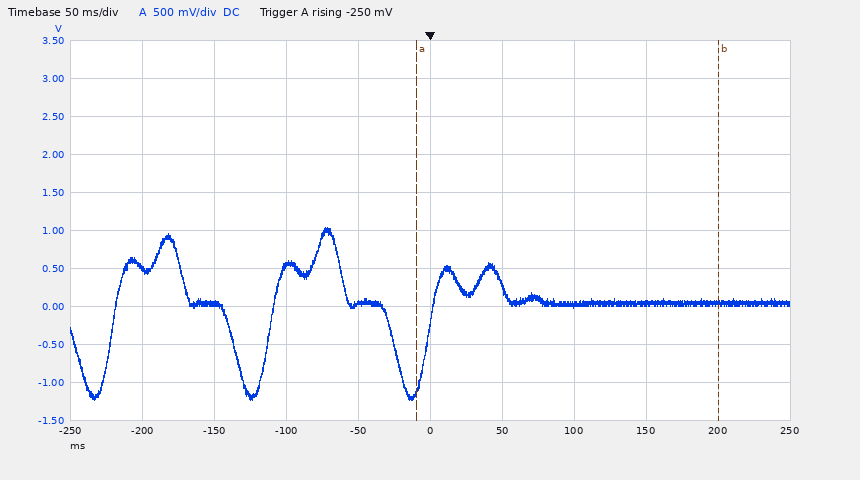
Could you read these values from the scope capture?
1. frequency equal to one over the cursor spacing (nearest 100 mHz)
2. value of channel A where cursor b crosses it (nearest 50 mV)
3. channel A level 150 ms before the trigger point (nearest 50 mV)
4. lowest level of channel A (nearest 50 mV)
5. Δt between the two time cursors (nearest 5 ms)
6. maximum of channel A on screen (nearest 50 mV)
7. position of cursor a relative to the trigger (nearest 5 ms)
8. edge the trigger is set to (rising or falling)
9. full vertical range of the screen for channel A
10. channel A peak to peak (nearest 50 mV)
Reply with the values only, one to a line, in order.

4.8 Hz
50 mV
50 mV
-1.25 V
210 ms
1.05 V
-10 ms
rising
5 V
2.30 V
